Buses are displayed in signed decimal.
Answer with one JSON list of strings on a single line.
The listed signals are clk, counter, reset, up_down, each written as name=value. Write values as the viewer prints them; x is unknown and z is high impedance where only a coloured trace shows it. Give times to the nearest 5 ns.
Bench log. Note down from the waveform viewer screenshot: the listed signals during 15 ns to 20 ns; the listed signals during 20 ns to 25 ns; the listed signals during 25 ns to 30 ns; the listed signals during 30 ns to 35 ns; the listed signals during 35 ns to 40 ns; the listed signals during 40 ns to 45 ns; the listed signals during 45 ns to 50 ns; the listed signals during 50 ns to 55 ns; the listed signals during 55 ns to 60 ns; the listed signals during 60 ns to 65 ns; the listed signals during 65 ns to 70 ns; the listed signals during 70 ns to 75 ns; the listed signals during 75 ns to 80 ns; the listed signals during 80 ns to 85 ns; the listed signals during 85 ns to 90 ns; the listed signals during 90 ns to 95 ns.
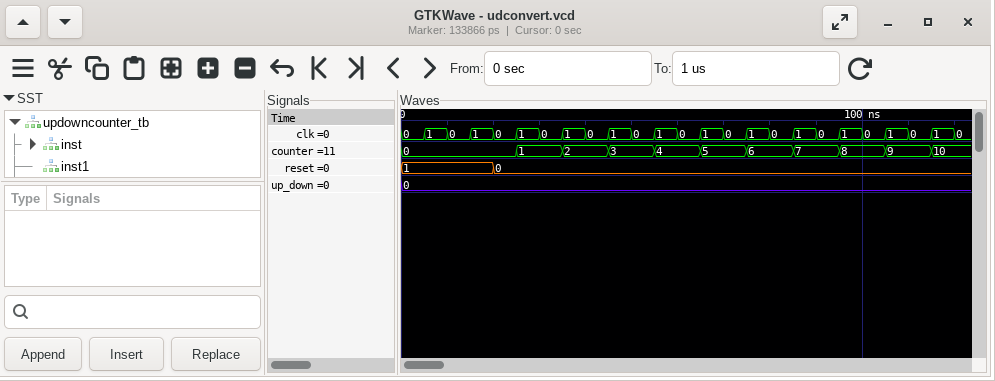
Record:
["clk=1, counter=0, reset=1, up_down=0", "clk=0, counter=0, reset=0, up_down=0", "clk=1, counter=1, reset=0, up_down=0", "clk=0, counter=1, reset=0, up_down=0", "clk=1, counter=2, reset=0, up_down=0", "clk=0, counter=2, reset=0, up_down=0", "clk=1, counter=3, reset=0, up_down=0", "clk=0, counter=3, reset=0, up_down=0", "clk=1, counter=4, reset=0, up_down=0", "clk=0, counter=4, reset=0, up_down=0", "clk=1, counter=5, reset=0, up_down=0", "clk=0, counter=5, reset=0, up_down=0", "clk=1, counter=6, reset=0, up_down=0", "clk=0, counter=6, reset=0, up_down=0", "clk=1, counter=7, reset=0, up_down=0", "clk=0, counter=7, reset=0, up_down=0"]
